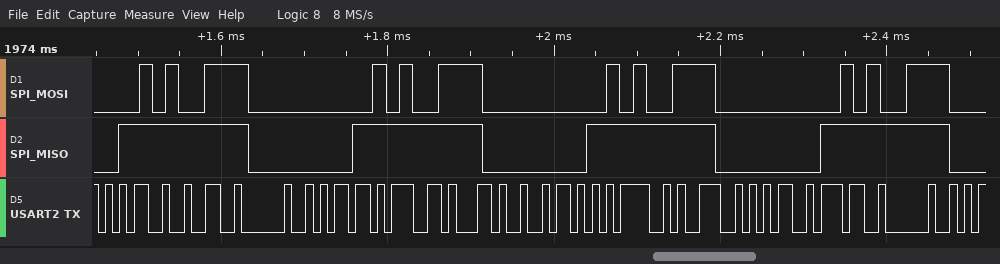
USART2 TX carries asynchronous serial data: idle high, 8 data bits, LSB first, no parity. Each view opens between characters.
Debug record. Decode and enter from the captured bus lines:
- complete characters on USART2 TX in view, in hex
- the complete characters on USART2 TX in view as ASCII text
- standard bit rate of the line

35, 32, 20, 6D, 67, 2C, 5A, 3D, 39, 35, 37, 20
"52 mg,Z=957 "
115200 baud
